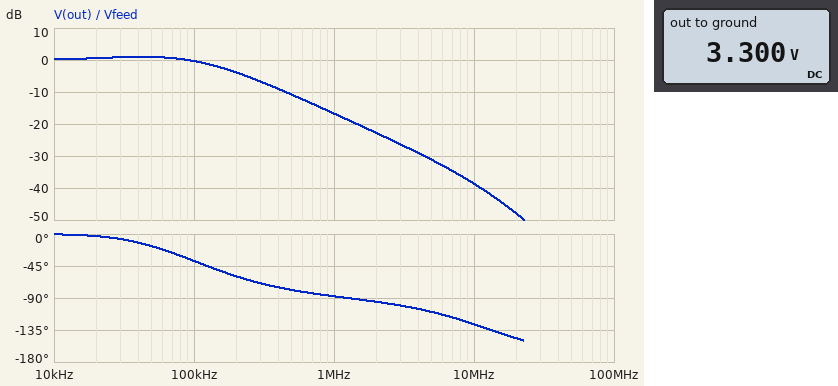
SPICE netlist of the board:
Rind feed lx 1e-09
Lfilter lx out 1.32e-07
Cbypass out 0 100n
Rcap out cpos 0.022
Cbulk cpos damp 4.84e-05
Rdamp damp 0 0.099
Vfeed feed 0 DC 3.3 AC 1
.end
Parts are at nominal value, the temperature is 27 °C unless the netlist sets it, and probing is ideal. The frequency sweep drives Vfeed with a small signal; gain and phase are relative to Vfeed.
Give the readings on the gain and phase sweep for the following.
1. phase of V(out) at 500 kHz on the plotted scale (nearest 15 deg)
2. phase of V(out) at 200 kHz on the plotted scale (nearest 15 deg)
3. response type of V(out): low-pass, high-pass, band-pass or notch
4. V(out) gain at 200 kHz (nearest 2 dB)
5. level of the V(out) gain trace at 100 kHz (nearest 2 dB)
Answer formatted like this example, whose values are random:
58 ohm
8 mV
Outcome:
-75 deg
-60 deg
low-pass
-4 dB
0 dB
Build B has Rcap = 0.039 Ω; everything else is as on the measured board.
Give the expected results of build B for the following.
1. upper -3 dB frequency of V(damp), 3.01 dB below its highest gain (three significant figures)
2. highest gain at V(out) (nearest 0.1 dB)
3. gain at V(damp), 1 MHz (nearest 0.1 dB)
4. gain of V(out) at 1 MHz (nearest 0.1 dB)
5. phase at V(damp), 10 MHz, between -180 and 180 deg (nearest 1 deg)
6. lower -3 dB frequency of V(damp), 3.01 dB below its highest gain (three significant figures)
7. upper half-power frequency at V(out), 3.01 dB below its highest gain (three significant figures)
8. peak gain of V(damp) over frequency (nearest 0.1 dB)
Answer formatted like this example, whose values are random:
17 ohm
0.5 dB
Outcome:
189 kHz
0.8 dB
-18.5 dB
-15.6 dB
-130 deg
21.2 kHz
165 kHz
-2.9 dB
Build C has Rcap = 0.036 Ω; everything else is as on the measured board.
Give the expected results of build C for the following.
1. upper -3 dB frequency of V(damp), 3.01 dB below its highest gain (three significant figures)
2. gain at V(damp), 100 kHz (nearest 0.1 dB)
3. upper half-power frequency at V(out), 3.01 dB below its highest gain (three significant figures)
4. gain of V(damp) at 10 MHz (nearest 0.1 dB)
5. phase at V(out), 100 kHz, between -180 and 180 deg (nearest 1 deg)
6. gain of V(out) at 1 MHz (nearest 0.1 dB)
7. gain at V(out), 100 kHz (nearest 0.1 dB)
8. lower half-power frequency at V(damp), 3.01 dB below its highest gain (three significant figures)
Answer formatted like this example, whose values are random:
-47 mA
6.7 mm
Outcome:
186 kHz
-3.2 dB
162 kHz
-40.8 dB
-34 deg
-15.8 dB
-0.3 dB
21.6 kHz
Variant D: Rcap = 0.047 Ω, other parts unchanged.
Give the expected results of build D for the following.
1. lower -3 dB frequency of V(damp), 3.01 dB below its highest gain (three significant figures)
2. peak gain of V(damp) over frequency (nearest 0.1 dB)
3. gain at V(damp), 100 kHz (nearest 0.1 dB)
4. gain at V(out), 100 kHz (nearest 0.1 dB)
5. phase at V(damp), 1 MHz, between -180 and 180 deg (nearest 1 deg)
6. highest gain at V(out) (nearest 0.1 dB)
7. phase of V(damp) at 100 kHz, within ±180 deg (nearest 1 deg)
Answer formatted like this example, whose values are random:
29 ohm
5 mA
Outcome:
20.3 kHz
-3.4 dB
-3.8 dB
-0.2 dB
-85 deg
0.7 dB
-19 deg
